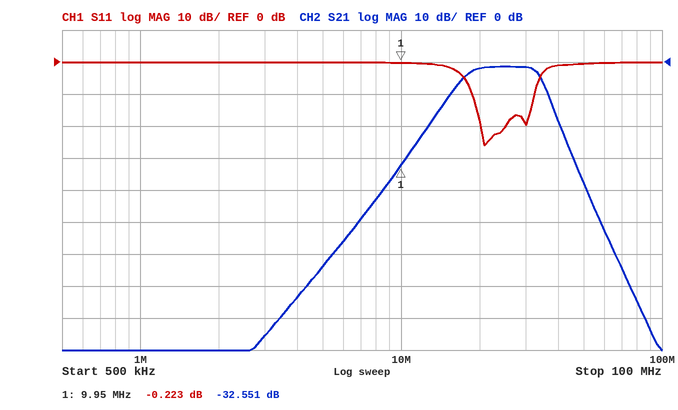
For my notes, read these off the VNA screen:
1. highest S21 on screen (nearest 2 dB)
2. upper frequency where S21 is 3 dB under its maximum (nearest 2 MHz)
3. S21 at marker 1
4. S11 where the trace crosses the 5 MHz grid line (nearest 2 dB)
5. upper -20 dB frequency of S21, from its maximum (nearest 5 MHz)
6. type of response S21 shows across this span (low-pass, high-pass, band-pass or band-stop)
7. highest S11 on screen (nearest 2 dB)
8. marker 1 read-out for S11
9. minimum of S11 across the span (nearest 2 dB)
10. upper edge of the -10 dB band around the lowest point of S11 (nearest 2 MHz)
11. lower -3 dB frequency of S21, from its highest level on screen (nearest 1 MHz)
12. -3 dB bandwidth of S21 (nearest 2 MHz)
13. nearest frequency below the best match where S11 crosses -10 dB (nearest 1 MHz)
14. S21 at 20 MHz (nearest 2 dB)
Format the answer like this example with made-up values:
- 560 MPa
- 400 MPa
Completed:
- -2 dB
- 34 MHz
- -32.551 dB
- 0 dB
- 40 MHz
- band-pass
- 0 dB
- -0.223 dB
- -26 dB
- 32 MHz
- 18 MHz
- 16 MHz
- 19 MHz
- -2 dB
